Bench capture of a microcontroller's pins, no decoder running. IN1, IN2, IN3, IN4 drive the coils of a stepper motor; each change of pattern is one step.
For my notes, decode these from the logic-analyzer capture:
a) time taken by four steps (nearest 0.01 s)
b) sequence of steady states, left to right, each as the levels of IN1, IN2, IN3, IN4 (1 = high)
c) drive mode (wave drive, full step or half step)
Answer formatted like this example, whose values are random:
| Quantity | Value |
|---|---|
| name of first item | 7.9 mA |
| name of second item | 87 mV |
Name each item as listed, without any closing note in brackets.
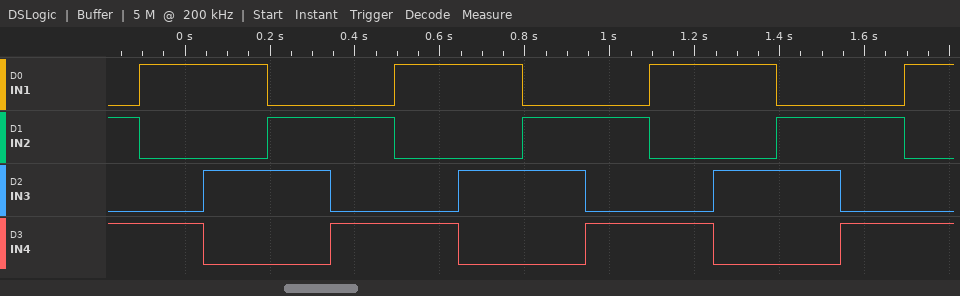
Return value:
| Quantity | Value |
|---|---|
| time taken by four steps | 0.60 s |
| sequence of steady states, left to right, each as the levels of IN1, IN2, IN3, IN4 | 0101 1001 1010 0110 0101 1001 1010 0110 0101 1001 1010 0110 0101 1001 |
| drive mode | full step |
